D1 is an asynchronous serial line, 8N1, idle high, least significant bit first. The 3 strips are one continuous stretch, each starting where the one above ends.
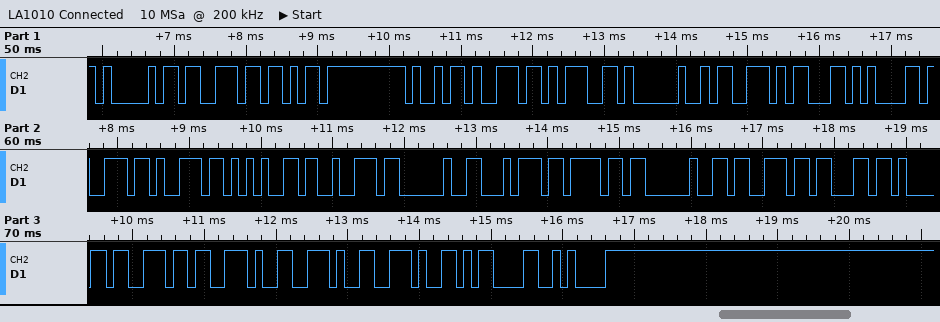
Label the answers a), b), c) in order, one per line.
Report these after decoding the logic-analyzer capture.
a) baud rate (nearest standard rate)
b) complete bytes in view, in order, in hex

a) 9600 baud
b) 41 73 6B 69 6E 67 20 73 63 61 6E 6E 65 72 20 74 6F 20 73 63 61 6E 2E 2E 2E 0D 0A
